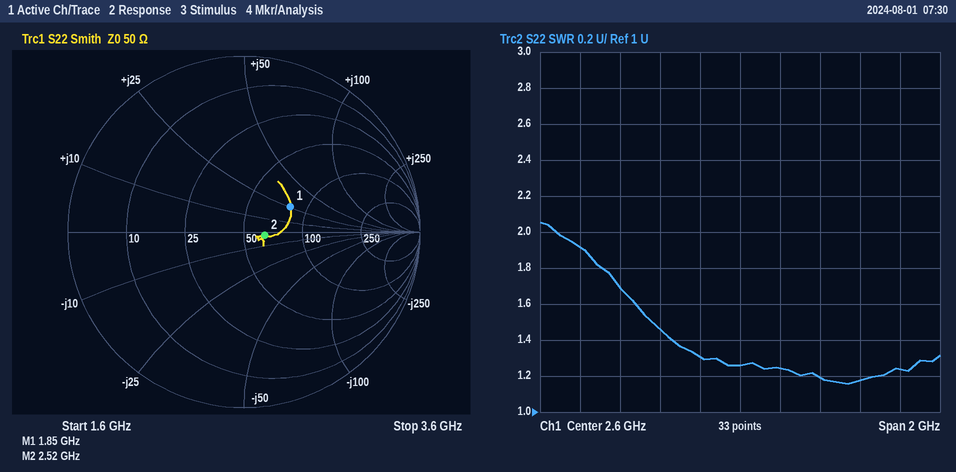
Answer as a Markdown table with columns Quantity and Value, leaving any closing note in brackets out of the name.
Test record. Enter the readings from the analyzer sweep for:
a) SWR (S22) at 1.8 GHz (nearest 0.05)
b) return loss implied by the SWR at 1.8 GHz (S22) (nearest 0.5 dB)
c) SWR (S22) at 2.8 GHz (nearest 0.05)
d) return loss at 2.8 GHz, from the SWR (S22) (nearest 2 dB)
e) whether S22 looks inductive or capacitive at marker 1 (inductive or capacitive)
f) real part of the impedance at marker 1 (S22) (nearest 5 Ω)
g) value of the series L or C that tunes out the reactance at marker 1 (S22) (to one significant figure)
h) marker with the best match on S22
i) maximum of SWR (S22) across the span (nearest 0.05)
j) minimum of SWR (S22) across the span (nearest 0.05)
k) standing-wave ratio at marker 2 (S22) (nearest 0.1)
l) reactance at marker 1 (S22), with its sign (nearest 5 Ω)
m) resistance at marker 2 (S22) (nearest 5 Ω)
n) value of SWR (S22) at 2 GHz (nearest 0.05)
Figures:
| Quantity | Value |
|---|---|
| SWR (S22) at 1.8 GHz | 1.90 |
| return loss implied by the SWR at 1.8 GHz (S22) | 10.0 dB |
| SWR (S22) at 2.8 GHz | 1.25 |
| return loss at 2.8 GHz, from the SWR (S22) | 20 dB |
| whether S22 looks inductive or capacitive at marker 1 | inductive |
| real part of the impedance at marker 1 (S22) | 80 Ω |
| value of the series L or C that tunes out the reactance at marker 1 (S22) | 3 pF |
| marker with the best match on S22 | marker 2 |
| maximum of SWR (S22) across the span | 2.05 |
| minimum of SWR (S22) across the span | 1.15 |
| standing-wave ratio at marker 2 (S22) | 1.3 |
| reactance at marker 1 (S22), with its sign | +25 Ω |
| resistance at marker 2 (S22) | 65 Ω |
| value of SWR (S22) at 2 GHz | 1.70 |
